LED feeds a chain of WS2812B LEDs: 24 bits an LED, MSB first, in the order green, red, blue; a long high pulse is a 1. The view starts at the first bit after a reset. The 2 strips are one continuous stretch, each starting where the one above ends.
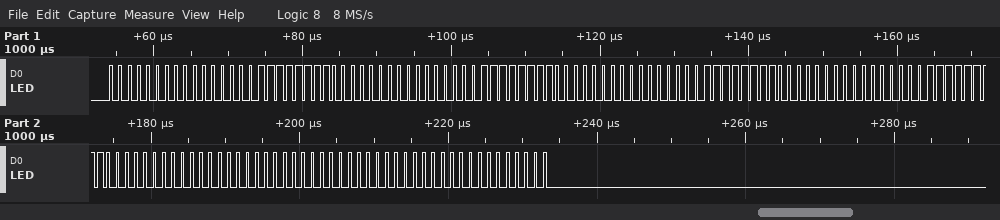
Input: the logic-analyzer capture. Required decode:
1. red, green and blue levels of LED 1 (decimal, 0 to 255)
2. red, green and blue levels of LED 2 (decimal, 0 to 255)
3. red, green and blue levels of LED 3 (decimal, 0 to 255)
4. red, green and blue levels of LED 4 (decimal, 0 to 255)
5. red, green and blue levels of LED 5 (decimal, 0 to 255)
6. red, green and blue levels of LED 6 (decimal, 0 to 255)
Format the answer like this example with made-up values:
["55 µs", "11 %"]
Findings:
["0, 0, 255", "0, 0, 255", "0, 0, 255", "0, 0, 255", "0, 0, 0", "0, 0, 0"]
